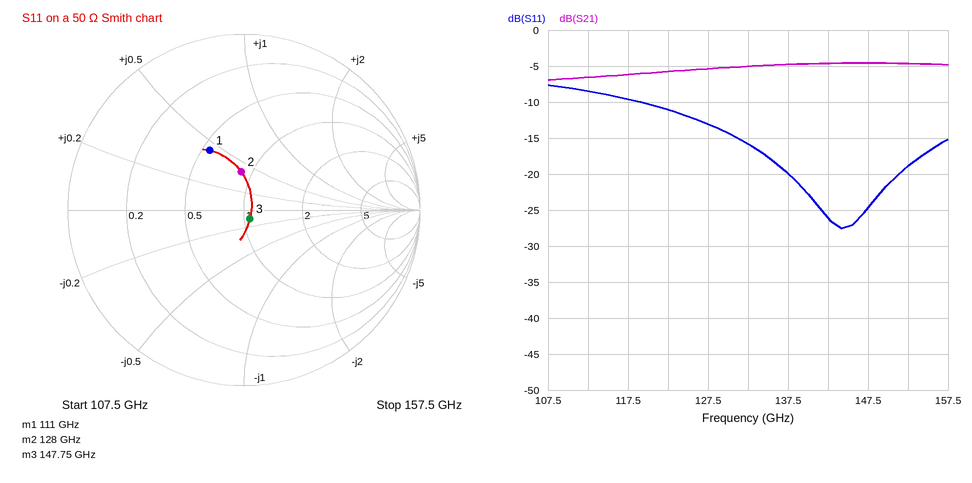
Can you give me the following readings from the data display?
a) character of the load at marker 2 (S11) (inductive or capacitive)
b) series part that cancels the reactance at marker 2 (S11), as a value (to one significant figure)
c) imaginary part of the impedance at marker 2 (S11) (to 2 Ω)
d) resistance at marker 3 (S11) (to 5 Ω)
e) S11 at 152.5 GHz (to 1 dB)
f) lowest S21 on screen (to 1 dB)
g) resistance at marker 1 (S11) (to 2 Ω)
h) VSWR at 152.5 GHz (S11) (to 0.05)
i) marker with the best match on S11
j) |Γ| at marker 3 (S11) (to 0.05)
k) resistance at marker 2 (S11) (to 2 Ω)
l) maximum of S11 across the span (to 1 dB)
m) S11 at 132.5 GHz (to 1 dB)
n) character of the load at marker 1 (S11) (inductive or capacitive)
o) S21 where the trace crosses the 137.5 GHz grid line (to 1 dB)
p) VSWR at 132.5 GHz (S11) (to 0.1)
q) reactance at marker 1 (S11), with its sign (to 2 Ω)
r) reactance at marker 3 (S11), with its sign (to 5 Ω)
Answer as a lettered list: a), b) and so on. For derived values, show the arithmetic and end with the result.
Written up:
a) inductive
b) C = 1/(2π × 128 GHz × 20 Ω) ≈ 62.2 fF, so 60 fF to one significant figure
c) +20 Ω
d) 55 Ω
e) -19 dB
f) -7 dB
g) 28 Ω
h) |Γ| = 10^(-19/20) = 0.1122; VSWR = (1 + 0.1122)/(1 − 0.1122) ≈ 1.25
i) marker 3
j) 0.05
k) 44 Ω
l) -8 dB
m) -16 dB
n) inductive
o) -5 dB
p) |Γ| = 10^(-16/20) = 0.1585; VSWR = (1 + 0.1585)/(1 − 0.1585) ≈ 1.4
q) +22 Ω
r) -5 Ω
